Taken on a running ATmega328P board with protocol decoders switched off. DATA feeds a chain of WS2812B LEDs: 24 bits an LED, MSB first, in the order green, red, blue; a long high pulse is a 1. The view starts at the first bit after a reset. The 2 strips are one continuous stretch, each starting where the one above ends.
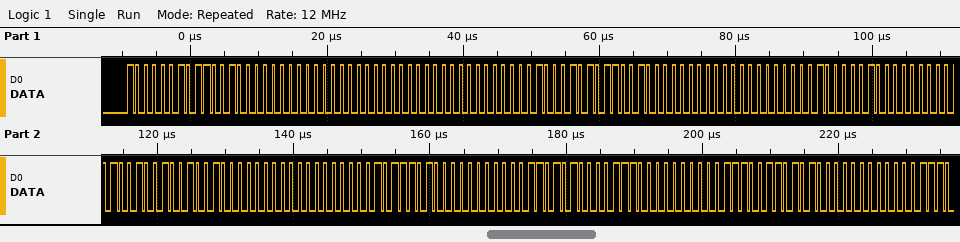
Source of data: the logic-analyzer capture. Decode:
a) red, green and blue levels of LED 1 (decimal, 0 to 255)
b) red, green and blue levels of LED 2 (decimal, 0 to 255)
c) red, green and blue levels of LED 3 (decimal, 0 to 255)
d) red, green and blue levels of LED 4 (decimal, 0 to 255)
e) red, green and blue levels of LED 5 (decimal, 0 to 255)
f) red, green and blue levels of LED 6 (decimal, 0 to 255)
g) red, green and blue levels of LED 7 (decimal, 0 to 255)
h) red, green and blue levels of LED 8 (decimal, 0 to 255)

200, 130, 0
0, 0, 0
200, 138, 0
65, 0, 0
146, 36, 0
93, 0, 0
135, 26, 0
168, 57, 0
